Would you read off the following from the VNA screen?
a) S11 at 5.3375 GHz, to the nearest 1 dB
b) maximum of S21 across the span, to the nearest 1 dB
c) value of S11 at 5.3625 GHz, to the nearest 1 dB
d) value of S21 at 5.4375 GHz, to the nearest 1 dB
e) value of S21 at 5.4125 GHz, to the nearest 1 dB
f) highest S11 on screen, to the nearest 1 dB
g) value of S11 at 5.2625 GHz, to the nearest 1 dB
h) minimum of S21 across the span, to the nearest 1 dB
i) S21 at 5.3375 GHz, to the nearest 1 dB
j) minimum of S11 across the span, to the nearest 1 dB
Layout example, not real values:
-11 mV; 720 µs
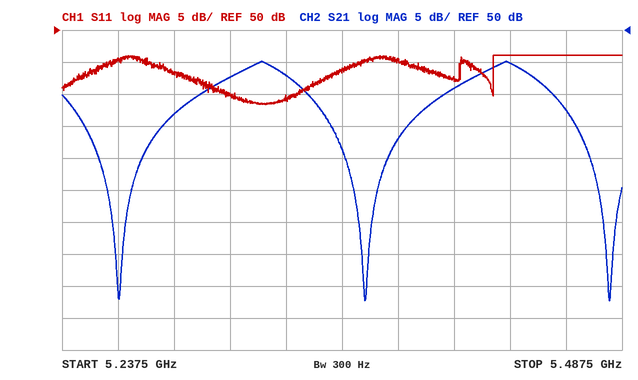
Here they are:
39 dB; 45 dB; 44 dB; 45 dB; 41 dB; 46 dB; 45 dB; 8 dB; 43 dB; 38 dB
